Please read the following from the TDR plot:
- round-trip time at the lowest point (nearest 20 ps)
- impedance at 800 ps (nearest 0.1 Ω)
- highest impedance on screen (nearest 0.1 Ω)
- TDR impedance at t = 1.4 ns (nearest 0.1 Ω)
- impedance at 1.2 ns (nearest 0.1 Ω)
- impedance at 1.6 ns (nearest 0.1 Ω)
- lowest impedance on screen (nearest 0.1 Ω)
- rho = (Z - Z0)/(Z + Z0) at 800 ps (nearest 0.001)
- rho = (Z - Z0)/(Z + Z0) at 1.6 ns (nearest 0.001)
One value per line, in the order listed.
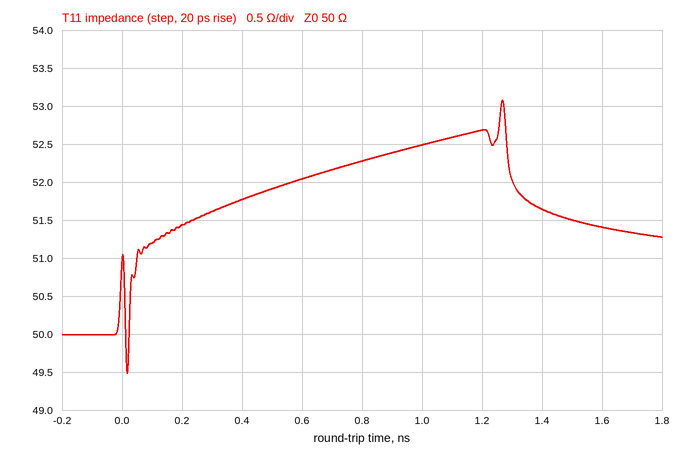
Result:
20 ps
52.3 Ω
53.1 Ω
51.6 Ω
52.7 Ω
51.4 Ω
49.5 Ω
+0.022
+0.014
